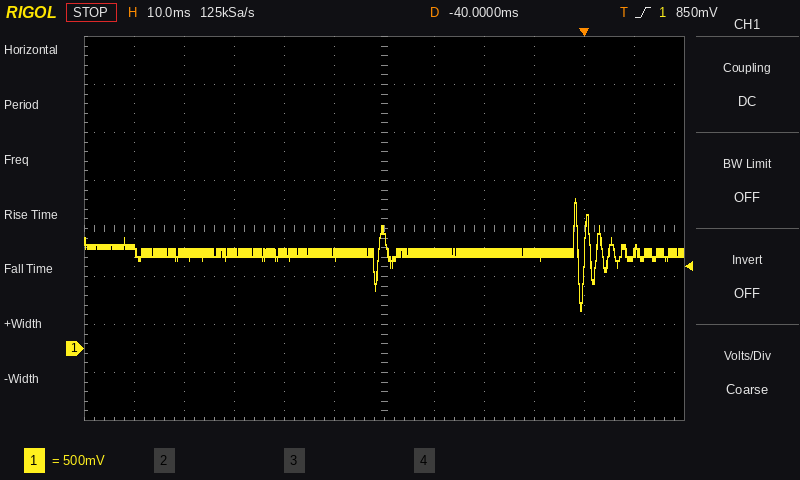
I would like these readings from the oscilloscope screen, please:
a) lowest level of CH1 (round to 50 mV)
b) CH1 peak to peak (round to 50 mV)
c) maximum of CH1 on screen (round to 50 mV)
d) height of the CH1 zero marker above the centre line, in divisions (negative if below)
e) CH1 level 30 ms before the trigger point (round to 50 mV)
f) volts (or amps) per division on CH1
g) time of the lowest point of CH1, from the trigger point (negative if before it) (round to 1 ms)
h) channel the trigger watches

400 mV
1.15 V
1.55 V
-2.5 div
1.00 V
500 mV
-1 ms
CH1
